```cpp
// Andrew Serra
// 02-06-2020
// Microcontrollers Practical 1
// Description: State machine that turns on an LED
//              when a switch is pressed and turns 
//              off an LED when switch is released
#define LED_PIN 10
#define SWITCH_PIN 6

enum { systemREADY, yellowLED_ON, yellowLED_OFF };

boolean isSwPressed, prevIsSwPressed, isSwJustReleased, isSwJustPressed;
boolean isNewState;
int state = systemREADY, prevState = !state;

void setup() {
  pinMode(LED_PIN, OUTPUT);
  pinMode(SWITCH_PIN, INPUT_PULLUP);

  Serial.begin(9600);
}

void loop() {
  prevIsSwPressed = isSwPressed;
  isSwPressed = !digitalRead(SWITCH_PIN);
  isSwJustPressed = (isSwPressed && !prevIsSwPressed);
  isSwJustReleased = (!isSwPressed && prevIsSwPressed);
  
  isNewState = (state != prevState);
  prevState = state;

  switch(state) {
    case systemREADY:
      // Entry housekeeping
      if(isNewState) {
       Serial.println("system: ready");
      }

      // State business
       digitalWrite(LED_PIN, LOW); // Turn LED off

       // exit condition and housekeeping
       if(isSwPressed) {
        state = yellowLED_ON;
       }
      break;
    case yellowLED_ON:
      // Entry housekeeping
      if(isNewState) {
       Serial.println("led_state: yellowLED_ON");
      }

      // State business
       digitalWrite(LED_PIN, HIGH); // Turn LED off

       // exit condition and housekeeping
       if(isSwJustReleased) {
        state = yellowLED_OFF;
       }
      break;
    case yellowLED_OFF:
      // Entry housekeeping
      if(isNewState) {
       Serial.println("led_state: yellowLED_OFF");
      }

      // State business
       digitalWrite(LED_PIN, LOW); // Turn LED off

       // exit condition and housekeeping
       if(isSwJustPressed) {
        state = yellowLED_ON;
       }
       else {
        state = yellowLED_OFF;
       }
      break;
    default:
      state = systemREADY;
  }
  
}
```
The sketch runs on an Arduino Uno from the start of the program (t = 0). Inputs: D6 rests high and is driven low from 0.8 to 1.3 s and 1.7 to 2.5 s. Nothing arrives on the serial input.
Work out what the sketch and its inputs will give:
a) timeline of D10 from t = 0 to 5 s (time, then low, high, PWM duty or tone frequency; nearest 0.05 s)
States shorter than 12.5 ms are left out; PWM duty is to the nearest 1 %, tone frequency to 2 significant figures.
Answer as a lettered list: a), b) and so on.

a) 0 s low; 0.8 s high; 1.3 s low; 1.7 s high; 2.5 s low
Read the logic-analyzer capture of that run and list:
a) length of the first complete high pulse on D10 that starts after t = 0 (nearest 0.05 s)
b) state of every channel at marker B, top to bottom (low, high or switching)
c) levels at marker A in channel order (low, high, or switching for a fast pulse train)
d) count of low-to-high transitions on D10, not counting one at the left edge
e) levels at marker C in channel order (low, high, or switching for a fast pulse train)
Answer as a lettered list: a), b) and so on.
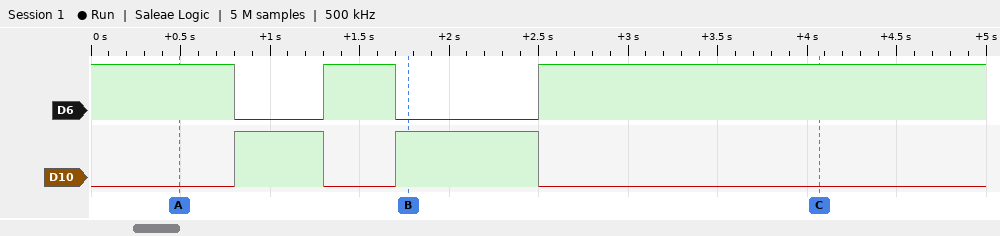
a) 0.50 s
b) D6 low, D10 high
c) D6 high, D10 low
d) 2
e) D6 high, D10 low
